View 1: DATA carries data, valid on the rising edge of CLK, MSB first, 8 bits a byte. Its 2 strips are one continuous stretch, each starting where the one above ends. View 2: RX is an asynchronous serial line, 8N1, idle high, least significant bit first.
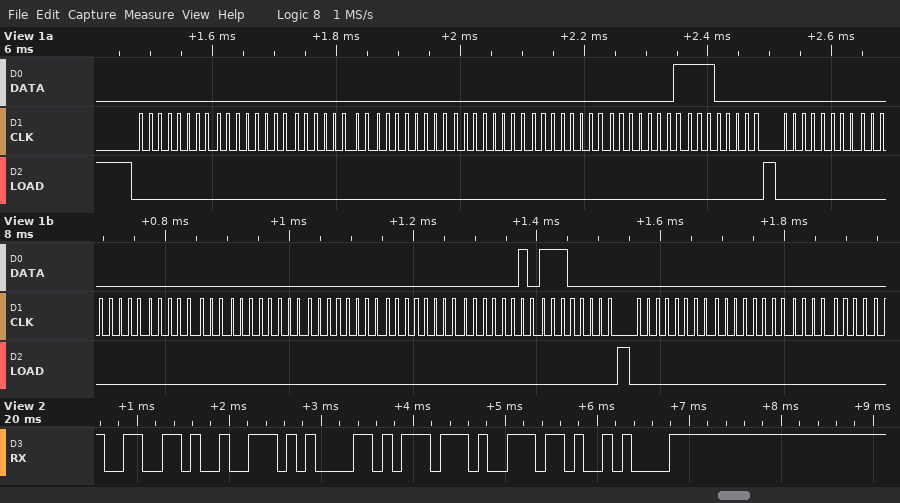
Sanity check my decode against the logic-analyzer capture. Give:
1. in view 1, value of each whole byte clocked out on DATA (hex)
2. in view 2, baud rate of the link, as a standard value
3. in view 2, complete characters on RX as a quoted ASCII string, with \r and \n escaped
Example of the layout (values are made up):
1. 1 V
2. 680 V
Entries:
1. 00 00 00 00 00 00 01 E0 00 00 00 00 00 00 02 E0 00 00 00
2. 9600 baud
3. "frawn\n"
